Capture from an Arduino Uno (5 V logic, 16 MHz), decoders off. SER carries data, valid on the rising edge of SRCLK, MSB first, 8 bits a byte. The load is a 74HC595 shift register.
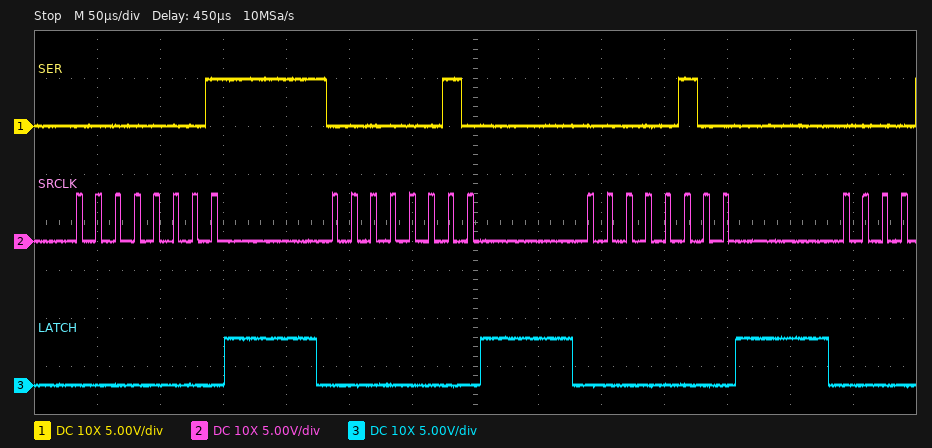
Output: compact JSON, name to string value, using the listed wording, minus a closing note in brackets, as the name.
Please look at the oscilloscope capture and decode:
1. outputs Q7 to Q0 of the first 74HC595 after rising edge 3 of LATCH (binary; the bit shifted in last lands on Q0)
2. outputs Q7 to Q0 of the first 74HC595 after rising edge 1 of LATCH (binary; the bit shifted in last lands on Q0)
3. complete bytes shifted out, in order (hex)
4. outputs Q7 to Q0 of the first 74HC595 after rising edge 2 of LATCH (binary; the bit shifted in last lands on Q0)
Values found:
{"outputs Q7 to Q0 of the first 74HC595 after rising edge 3 of LATCH": "00000100", "outputs Q7 to Q0 of the first 74HC595 after rising edge 1 of LATCH": "00000001", "complete bytes shifted out, in order": "0x01 0x02 0x04", "outputs Q7 to Q0 of the first 74HC595 after rising edge 2 of LATCH": "00000010"}
